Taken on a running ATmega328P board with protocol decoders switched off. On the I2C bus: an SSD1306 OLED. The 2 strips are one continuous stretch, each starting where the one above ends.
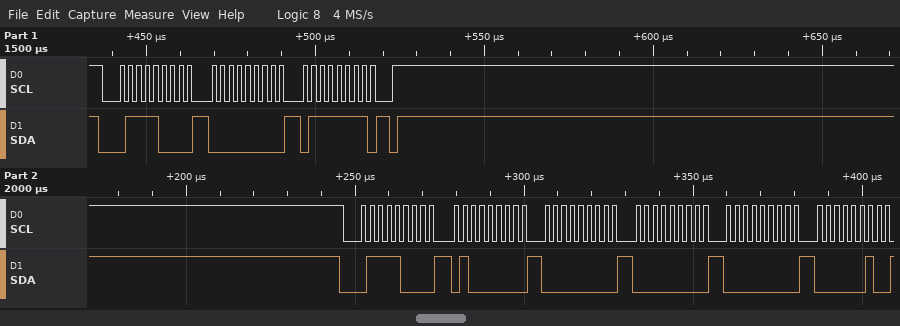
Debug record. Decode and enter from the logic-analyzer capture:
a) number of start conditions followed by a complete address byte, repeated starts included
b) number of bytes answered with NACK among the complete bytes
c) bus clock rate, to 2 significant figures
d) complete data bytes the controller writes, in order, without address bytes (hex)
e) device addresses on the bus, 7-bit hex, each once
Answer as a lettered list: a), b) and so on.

a) 2
b) 0
c) 400 kHz
d) 00 7F 40 00 00 00 02
e) 0x3C
